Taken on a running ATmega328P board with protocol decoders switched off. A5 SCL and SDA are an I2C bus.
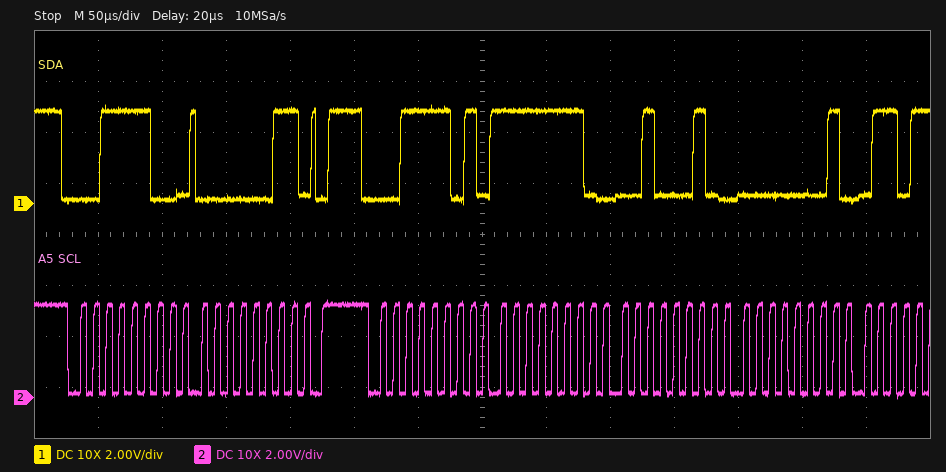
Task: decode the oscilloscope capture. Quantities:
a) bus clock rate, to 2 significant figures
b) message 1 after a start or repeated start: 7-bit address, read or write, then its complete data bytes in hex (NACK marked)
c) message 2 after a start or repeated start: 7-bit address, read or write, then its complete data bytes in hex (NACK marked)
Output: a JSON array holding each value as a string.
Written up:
["100 kHz", "0x1E write: 03", "0x1E read: FE 22 01"]
